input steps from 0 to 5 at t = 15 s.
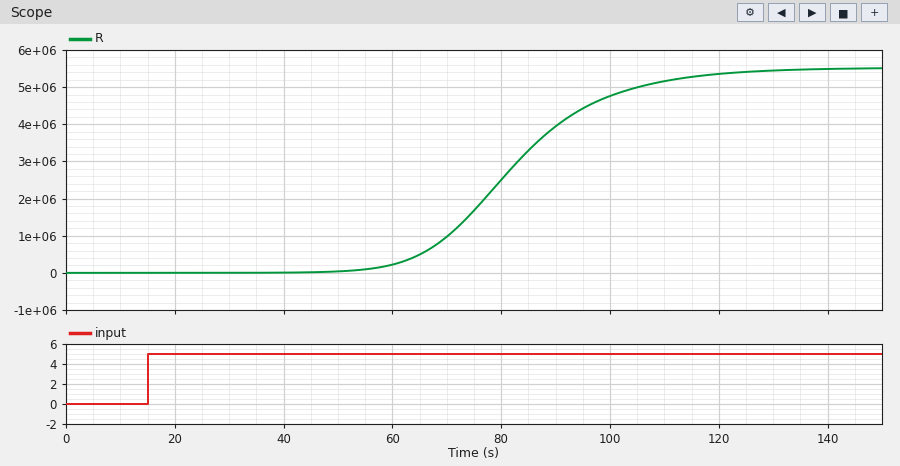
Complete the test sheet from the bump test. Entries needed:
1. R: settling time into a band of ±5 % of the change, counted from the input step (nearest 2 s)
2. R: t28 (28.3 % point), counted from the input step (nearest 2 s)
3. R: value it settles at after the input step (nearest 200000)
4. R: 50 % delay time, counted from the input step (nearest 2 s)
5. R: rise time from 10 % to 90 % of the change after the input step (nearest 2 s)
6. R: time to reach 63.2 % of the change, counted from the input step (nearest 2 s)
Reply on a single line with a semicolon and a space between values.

98 s; 60 s; 5600000; 66 s; 38 s; 72 s
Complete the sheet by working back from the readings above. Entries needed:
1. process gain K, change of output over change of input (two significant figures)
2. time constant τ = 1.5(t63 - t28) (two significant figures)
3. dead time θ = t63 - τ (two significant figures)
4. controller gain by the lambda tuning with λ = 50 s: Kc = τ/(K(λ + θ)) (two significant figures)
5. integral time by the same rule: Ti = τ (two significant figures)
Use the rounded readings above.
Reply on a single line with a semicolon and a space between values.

1100000; 18 s; 54 s; 0.00000016; 18 s
